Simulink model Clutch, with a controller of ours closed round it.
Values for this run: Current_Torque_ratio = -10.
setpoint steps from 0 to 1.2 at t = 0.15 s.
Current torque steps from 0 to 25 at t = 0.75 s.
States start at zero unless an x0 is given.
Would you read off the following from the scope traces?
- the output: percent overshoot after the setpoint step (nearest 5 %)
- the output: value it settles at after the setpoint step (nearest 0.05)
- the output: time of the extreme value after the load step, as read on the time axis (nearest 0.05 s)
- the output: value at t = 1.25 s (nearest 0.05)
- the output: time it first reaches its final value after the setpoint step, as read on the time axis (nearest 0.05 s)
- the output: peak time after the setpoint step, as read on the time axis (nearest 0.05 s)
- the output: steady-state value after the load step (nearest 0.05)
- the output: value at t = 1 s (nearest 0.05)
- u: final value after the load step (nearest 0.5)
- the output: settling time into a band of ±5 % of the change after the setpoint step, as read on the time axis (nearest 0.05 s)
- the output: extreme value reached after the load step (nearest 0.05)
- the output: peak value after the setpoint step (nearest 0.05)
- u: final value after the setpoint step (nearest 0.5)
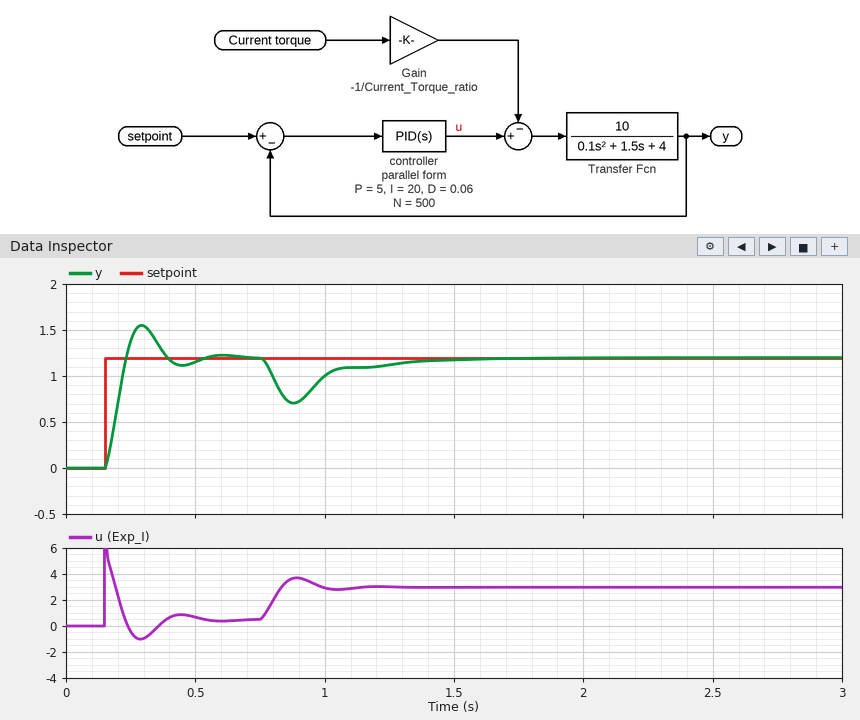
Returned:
30 %
1.20
0.90 s
1.10
0.25 s
0.30 s
1.20
1.00
3.0
0.50 s
0.70
1.55
0.5
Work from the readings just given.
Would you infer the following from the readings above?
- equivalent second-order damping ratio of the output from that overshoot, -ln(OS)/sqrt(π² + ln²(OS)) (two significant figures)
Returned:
0.36
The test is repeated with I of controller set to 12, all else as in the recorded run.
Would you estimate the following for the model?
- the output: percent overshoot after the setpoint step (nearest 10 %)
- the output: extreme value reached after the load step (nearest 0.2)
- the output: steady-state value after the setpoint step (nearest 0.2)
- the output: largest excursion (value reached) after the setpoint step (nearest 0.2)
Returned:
20 %
0.6
1.2
1.4
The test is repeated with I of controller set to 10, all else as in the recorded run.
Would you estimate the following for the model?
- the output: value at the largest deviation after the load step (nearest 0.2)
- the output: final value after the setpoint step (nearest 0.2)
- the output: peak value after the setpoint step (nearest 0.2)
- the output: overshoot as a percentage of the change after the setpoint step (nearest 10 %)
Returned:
0.6
1.2
1.4
20 %
